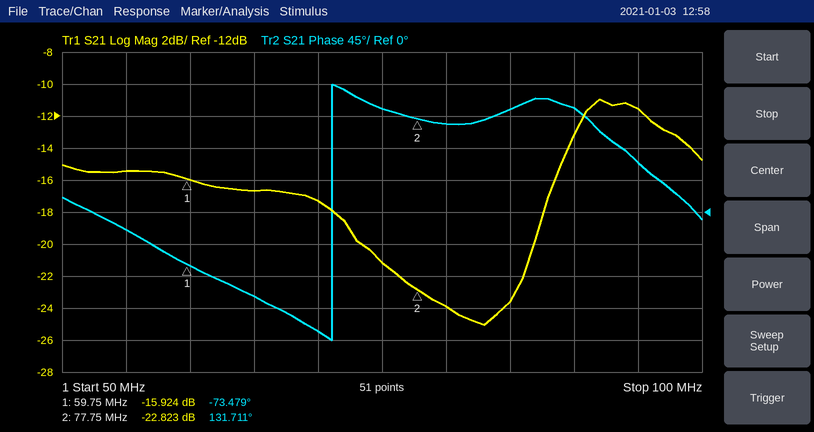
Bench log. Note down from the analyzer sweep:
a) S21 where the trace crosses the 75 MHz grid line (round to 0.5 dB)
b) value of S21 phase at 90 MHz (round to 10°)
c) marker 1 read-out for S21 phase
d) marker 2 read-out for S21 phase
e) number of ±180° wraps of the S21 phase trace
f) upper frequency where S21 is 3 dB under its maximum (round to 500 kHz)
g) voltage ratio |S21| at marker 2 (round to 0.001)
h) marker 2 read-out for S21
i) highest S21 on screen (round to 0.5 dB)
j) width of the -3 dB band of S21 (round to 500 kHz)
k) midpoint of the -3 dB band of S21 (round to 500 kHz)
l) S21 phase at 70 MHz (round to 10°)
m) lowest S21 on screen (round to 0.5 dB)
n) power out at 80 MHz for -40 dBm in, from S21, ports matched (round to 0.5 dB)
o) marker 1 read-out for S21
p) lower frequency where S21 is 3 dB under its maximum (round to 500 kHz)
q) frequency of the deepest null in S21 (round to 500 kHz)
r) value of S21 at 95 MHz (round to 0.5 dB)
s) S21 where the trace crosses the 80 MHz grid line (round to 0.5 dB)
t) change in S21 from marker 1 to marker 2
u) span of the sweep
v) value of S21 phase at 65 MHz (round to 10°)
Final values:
-21.0 dB
150°
-73.479°
131.711°
1
99.0 MHz
0.072
-22.823 dB
-11.0 dB
9.5 MHz
94.5 MHz
-170°
-25.0 dB
-64.0 dBm
-15.924 dB
89.5 MHz
83.0 MHz
-11.5 dB
-24.0 dB
-6.899 dB
50 MHz
-120°
